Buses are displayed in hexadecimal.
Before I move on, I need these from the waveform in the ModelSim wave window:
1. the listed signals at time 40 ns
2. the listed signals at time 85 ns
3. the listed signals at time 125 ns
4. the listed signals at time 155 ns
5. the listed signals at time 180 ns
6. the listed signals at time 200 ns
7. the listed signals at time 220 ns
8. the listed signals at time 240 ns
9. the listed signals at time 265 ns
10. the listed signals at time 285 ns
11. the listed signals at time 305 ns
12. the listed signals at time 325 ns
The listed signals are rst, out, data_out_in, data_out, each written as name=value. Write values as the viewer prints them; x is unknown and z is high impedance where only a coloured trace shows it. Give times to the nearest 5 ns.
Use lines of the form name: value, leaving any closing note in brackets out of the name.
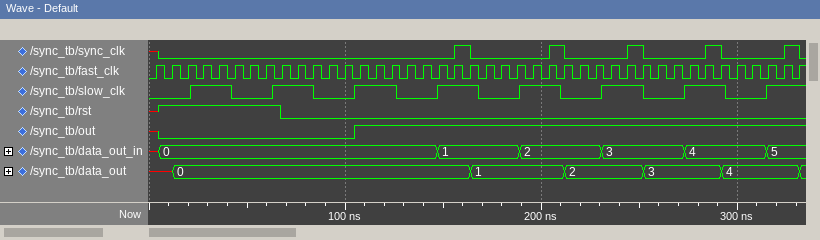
the listed signals at time 40 ns: rst=1, out=0, data_out_in=0, data_out=0
the listed signals at time 85 ns: rst=0, out=0, data_out_in=0, data_out=0
the listed signals at time 125 ns: rst=0, out=1, data_out_in=0, data_out=0
the listed signals at time 155 ns: rst=0, out=1, data_out_in=1, data_out=0
the listed signals at time 180 ns: rst=0, out=1, data_out_in=1, data_out=1
the listed signals at time 200 ns: rst=0, out=1, data_out_in=2, data_out=1
the listed signals at time 220 ns: rst=0, out=1, data_out_in=2, data_out=2
the listed signals at time 240 ns: rst=0, out=1, data_out_in=3, data_out=2
the listed signals at time 265 ns: rst=0, out=1, data_out_in=3, data_out=3
the listed signals at time 285 ns: rst=0, out=1, data_out_in=4, data_out=3
the listed signals at time 305 ns: rst=0, out=1, data_out_in=4, data_out=4
the listed signals at time 325 ns: rst=0, out=1, data_out_in=5, data_out=4
